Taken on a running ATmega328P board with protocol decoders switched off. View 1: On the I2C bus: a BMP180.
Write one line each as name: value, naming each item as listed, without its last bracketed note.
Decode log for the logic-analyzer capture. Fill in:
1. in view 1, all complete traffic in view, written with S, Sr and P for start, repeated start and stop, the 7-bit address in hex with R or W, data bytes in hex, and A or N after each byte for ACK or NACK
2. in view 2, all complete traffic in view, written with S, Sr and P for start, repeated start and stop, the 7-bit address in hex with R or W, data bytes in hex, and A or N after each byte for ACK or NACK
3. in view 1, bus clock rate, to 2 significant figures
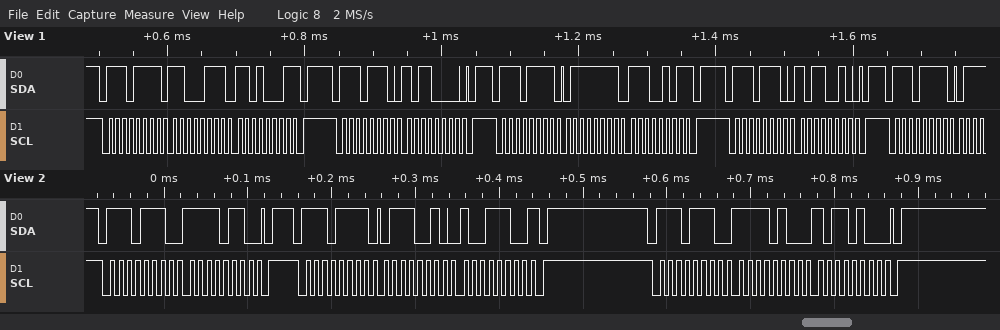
in view 1, all complete traffic in view, written with S, Sr and P for start, repeated start and stop, the 7-bit address in hex with R or W, data bytes in hex, and A or N after each byte for ACK or NACK: S 77R A C7 A D1 N P S 77W A B0 A P S 77R A 7F A E5 N P S 77W A B2 A P S 77R A
in view 2, all complete traffic in view, written with S, Sr and P for start, repeated start and stop, the 7-bit address in hex with R or W, data bytes in hex, and A or N after each byte for ACK or NACK: S 77W A F6 A P S 77R A 72 A 9C N P S 77W A F4 A B4 A P
in view 1, bus clock rate, to 2 significant figures: 100 kHz
